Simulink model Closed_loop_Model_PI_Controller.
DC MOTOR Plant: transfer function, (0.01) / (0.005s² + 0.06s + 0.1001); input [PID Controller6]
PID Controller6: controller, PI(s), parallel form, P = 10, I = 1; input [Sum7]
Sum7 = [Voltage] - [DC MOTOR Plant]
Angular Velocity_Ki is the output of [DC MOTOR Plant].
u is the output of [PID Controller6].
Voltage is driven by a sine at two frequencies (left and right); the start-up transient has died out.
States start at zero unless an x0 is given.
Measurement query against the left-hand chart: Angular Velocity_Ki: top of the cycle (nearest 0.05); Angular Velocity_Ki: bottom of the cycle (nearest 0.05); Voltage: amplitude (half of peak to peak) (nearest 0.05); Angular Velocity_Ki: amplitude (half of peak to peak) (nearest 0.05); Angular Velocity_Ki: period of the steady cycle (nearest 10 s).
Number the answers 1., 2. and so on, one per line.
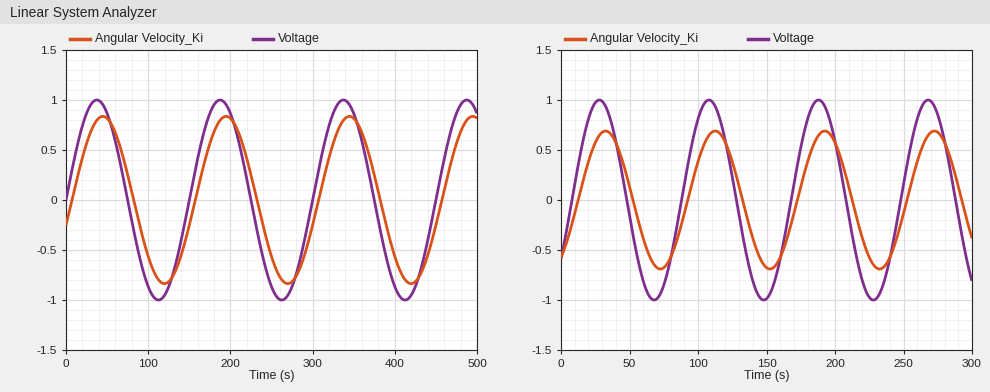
1. 0.85
2. -0.85
3. 1.00
4. 0.85
5. 150 s
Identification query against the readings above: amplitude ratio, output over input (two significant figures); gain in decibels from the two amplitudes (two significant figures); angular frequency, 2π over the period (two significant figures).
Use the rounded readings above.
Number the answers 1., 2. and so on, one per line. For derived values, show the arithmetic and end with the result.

1. 0.85 / 1 = 0.85
2. 20 log10(0.85 / 1) = -1.4 dB
3. 2π / 150 = 0.042 rad/s
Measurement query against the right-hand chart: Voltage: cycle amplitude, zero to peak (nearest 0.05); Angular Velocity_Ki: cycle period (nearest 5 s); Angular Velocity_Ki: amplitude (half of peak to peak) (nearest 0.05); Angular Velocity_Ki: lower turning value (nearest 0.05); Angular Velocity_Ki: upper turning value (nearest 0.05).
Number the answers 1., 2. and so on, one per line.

1. 1.00
2. 80 s
3. 0.70
4. -0.70
5. 0.70
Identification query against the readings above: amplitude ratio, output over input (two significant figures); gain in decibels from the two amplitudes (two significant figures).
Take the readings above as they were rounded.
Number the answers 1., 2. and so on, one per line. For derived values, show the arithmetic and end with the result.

1. 0.7 / 1 = 0.70
2. 20 log10(0.7 / 1) = -3.1 dB
